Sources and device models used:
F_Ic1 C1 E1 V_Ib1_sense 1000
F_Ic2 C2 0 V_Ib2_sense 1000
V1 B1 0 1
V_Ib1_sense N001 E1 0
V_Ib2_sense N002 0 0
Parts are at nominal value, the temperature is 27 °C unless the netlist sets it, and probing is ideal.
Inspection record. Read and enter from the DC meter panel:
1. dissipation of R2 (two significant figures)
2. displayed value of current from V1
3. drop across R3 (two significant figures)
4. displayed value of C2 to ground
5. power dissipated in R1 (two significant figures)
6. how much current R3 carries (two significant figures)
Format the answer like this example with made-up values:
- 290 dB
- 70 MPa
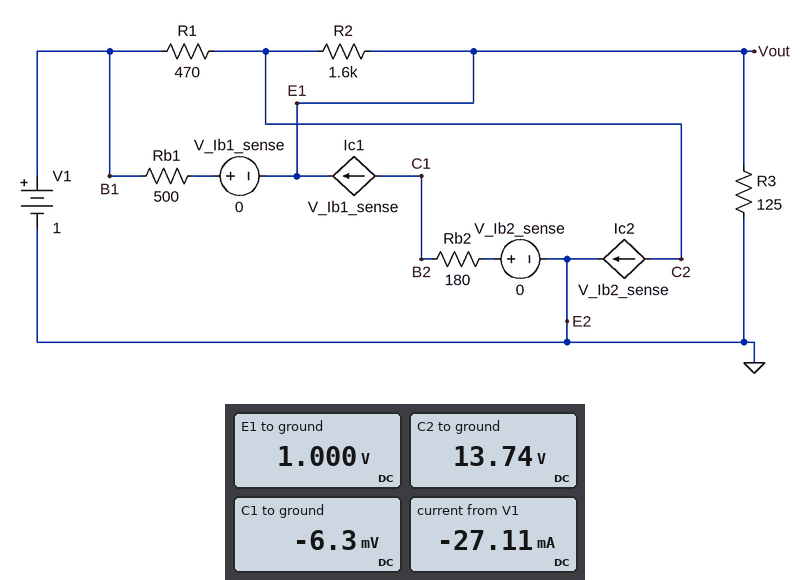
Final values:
- 100 mW
- -27.11 mA
- 1.0 V
- 13.74 V
- 350 mW
- 8.0 mA
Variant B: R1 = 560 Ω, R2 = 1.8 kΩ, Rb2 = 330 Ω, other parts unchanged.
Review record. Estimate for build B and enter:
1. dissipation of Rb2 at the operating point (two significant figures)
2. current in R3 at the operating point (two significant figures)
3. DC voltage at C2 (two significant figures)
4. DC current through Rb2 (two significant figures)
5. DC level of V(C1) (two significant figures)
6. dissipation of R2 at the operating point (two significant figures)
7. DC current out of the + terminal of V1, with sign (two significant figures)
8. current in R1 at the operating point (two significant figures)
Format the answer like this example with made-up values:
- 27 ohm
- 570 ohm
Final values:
- 370 nW
- 8.0 mA
- 15 V
- 34 µA
- -11 mV
- 110 mW
- -26 mA
- 26 mA
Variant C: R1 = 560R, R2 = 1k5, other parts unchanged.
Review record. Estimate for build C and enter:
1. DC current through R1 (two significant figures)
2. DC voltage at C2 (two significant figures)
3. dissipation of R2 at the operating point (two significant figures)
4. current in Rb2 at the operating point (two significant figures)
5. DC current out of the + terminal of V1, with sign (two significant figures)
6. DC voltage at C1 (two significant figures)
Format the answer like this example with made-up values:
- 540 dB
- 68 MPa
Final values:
- 21 mA
- 13 V
- 95 mW
- 29 µA
- -21 mA
- -5.3 mV
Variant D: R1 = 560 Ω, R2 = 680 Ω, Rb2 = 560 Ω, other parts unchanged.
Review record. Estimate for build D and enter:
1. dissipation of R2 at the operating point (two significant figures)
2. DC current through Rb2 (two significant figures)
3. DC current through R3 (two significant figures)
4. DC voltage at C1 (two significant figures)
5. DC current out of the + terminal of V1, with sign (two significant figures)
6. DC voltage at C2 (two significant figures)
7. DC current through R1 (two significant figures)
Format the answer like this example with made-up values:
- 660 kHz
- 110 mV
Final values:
- 43 mW
- 18 µA
- 8.0 mA
- -9.9 mV
- -9.7 mA
- 6.4 V
- 9.7 mA
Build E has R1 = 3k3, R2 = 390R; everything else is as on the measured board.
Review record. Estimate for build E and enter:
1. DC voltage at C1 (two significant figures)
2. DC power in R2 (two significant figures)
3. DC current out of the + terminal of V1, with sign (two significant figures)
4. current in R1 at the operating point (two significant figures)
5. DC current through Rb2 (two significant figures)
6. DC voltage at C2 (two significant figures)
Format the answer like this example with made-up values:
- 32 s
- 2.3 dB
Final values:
- -1.6 mV
- 25 mW
- -940 µA
- 940 µA
- 8.9 µA
- 4.1 V
